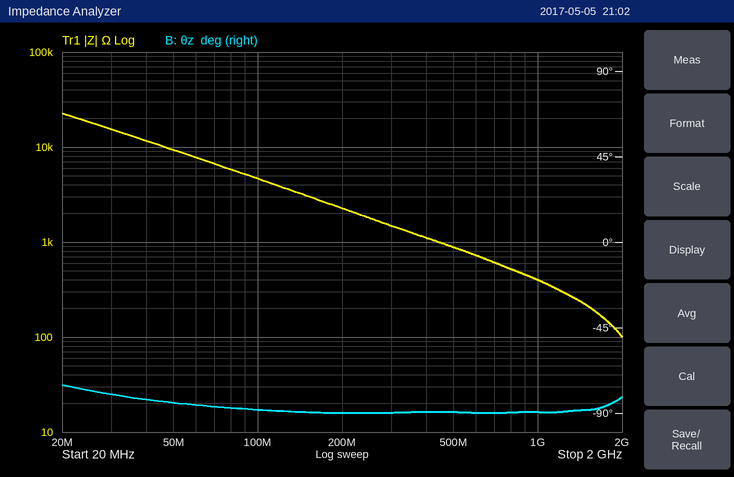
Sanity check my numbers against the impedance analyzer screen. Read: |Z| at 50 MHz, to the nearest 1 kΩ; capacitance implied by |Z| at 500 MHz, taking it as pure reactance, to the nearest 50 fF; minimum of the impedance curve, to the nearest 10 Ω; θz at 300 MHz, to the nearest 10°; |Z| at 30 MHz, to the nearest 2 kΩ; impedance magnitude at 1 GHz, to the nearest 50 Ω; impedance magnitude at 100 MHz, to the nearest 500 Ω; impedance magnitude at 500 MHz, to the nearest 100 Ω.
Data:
9 kΩ
350 fF
100 Ω
-90°
16 kΩ
400 Ω
4.5 kΩ
900 Ω
